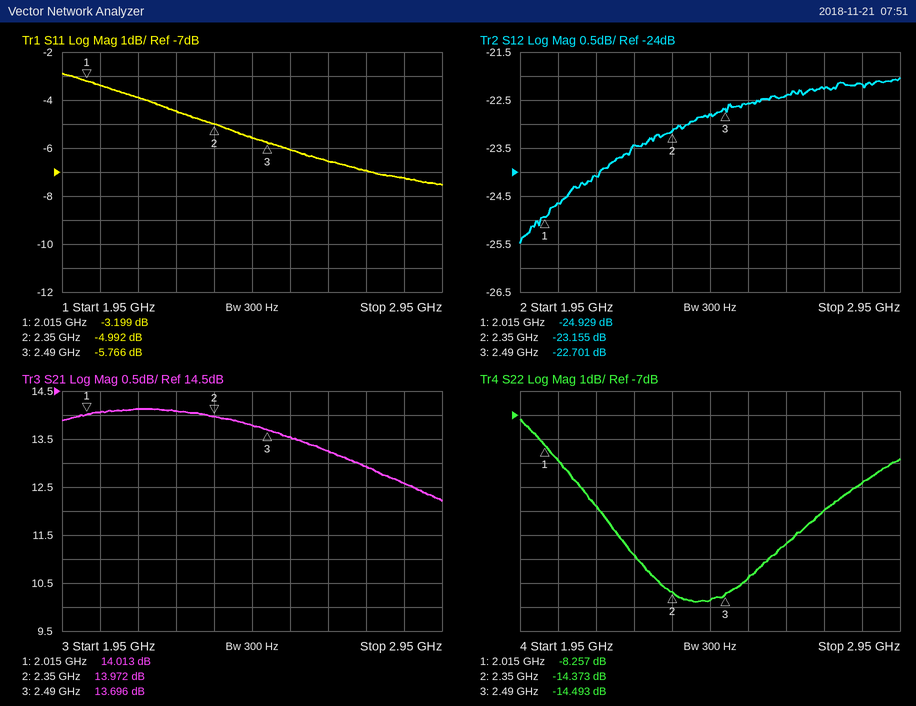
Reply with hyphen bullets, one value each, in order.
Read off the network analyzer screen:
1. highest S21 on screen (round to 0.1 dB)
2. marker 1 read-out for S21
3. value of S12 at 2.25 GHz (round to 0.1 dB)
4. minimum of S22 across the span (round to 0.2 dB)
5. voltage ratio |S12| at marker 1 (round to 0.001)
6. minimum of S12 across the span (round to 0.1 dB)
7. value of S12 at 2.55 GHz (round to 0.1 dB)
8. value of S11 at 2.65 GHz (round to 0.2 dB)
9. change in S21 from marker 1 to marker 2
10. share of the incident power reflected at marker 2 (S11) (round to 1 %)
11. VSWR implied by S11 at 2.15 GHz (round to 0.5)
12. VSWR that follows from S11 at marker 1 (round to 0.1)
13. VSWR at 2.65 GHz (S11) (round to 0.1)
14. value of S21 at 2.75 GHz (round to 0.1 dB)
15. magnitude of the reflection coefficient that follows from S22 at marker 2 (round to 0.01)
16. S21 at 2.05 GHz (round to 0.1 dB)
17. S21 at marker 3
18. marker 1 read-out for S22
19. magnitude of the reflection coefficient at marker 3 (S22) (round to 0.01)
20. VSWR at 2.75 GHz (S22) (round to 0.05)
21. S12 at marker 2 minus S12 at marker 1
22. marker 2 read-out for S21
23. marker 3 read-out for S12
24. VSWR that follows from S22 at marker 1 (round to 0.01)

- 14.1 dB
- 14.013 dB
- -23.4 dB
- -14.8 dB
- 0.057
- -25.5 dB
- -22.6 dB
- -6.6 dB
- -0.041 dB
- 32 %
- 4.5
- 5.5
- 2.8
- 12.9 dB
- 0.19
- 14.1 dB
- 13.696 dB
- -8.257 dB
- 0.19
- 1.80
- 1.774 dB
- 13.972 dB
- -22.701 dB
- 2.26
